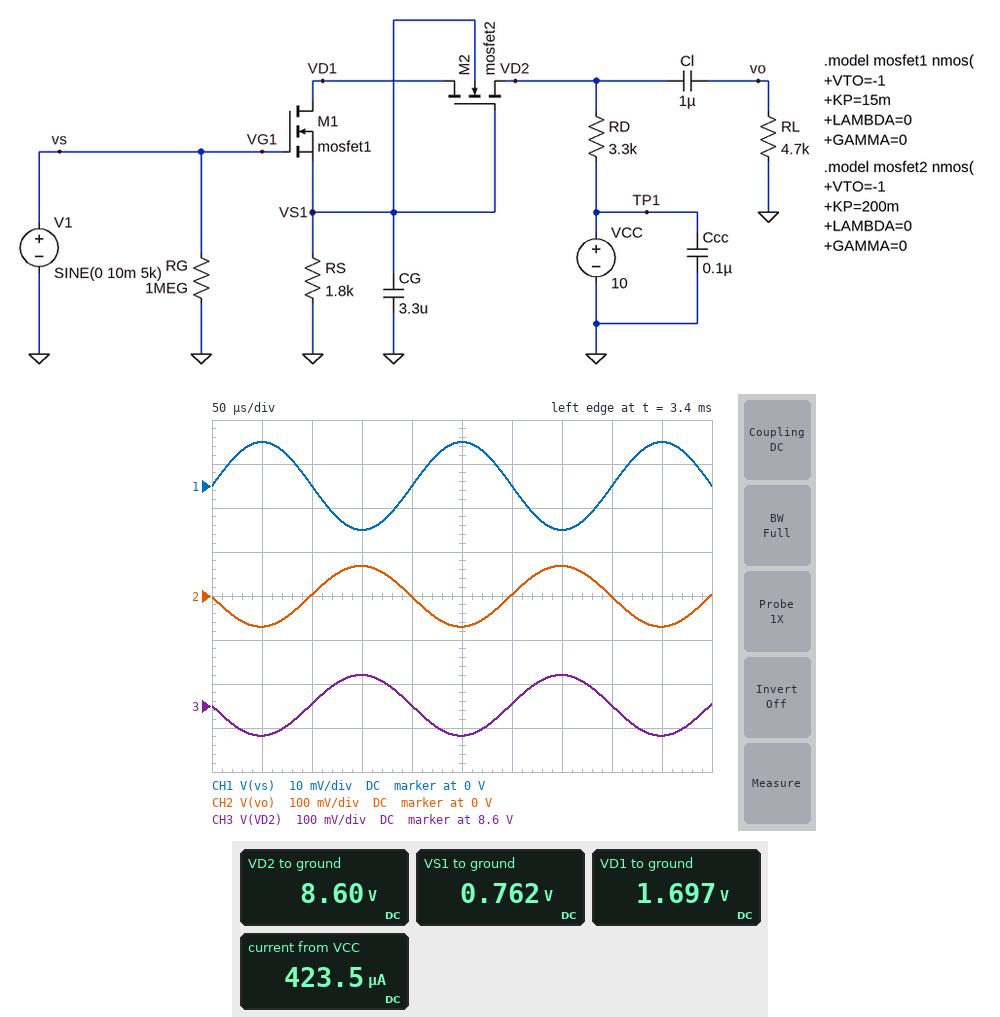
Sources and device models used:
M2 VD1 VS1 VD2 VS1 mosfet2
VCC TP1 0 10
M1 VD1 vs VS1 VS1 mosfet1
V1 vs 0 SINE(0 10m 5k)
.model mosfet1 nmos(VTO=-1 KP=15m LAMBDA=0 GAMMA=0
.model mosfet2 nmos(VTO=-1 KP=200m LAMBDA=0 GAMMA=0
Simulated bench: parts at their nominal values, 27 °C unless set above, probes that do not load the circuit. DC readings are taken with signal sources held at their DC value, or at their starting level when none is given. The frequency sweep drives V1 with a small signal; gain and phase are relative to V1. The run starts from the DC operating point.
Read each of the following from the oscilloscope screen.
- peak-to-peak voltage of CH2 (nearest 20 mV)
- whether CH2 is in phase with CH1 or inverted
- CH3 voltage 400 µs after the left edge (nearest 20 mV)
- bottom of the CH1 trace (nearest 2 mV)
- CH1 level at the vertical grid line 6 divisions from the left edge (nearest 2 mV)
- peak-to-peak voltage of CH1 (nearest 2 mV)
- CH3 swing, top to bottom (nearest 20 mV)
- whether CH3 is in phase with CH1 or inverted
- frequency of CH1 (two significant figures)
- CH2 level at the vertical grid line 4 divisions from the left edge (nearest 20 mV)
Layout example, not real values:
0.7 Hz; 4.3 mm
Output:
140 mV; inverted; 8.60 V; -10 mV; 0 V; 20 mV; 140 mV; inverted; 5.0 kHz; 0 V
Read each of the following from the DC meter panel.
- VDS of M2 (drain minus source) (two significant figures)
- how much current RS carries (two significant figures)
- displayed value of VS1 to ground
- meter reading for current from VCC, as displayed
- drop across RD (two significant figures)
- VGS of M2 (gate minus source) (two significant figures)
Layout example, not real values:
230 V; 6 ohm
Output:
-6.9 V; 420 µA; 0.762 V; 423.5 µA; 1.4 V; -7.8 V
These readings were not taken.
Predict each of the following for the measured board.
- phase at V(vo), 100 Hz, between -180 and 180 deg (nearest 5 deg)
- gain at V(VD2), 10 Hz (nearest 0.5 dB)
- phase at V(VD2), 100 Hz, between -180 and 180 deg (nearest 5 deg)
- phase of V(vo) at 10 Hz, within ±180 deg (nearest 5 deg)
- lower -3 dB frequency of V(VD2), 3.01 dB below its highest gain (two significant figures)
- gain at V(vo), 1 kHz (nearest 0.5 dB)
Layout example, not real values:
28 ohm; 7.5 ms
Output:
-120 deg; 4.0 dB; -140 deg; -100 deg; 190 Hz; 16.5 dB
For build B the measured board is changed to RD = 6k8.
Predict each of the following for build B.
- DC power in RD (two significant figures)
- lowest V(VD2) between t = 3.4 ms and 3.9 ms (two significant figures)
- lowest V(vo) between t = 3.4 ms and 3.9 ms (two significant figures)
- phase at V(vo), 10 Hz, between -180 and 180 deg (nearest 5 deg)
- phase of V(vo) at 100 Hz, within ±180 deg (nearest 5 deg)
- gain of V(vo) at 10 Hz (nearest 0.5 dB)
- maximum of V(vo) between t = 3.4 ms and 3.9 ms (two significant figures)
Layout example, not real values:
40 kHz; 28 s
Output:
1.2 mW; 7.0 V; -100 mV; -110 deg; -125 deg; -1.5 dB; 98 mV
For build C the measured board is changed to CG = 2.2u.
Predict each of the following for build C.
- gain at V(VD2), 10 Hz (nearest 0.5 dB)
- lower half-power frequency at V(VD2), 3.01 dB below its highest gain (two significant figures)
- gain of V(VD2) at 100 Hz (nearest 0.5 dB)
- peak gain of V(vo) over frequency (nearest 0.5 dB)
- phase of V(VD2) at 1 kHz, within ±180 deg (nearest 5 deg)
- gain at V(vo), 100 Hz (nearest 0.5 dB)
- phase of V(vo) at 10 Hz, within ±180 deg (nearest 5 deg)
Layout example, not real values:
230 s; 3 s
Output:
3.5 dB; 290 Hz; 8.0 dB; 17.0 dB; -165 deg; 7.5 dB; -105 deg
